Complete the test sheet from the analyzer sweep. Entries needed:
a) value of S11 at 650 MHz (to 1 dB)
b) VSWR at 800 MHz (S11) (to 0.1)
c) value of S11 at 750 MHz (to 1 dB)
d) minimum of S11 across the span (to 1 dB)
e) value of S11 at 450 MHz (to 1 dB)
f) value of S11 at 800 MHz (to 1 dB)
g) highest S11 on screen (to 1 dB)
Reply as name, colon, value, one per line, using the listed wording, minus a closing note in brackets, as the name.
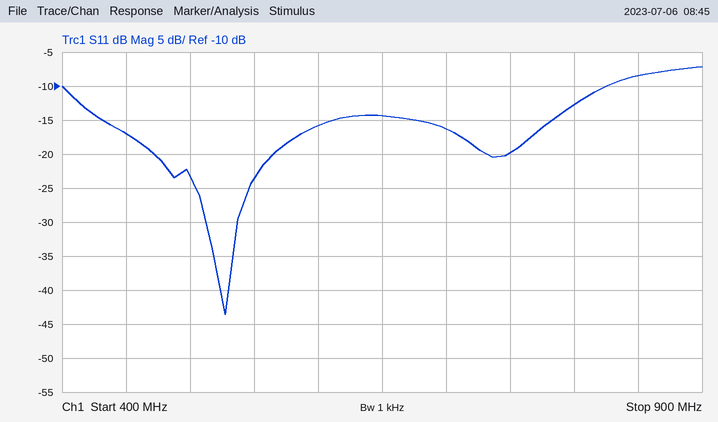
value of S11 at 650 MHz: -14 dB
VSWR at 800 MHz (S11): 1.6
value of S11 at 750 MHz: -20 dB
minimum of S11 across the span: -44 dB
value of S11 at 450 MHz: -17 dB
value of S11 at 800 MHz: -13 dB
highest S11 on screen: -7 dB
